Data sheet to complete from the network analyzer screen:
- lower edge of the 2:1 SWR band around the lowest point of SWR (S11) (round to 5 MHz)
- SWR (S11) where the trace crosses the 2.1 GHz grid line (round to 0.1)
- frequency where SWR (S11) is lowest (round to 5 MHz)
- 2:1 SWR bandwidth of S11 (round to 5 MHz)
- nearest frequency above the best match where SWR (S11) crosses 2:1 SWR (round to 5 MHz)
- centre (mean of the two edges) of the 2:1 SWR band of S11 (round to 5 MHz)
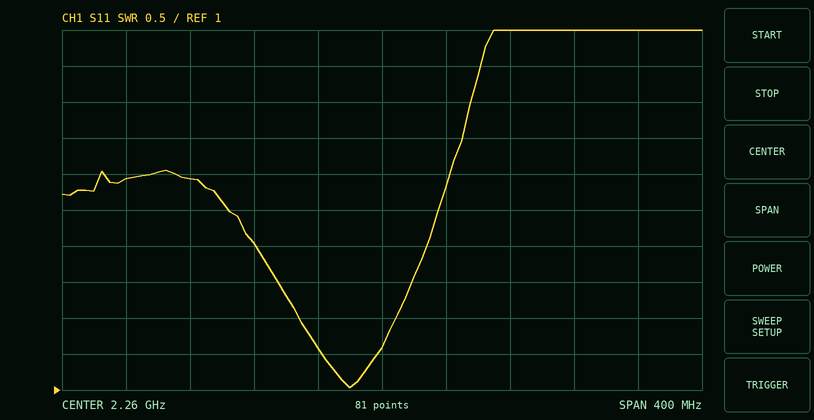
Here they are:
2.210 GHz
3.9
2.240 GHz
60 MHz
2.270 GHz
2.240 GHz
